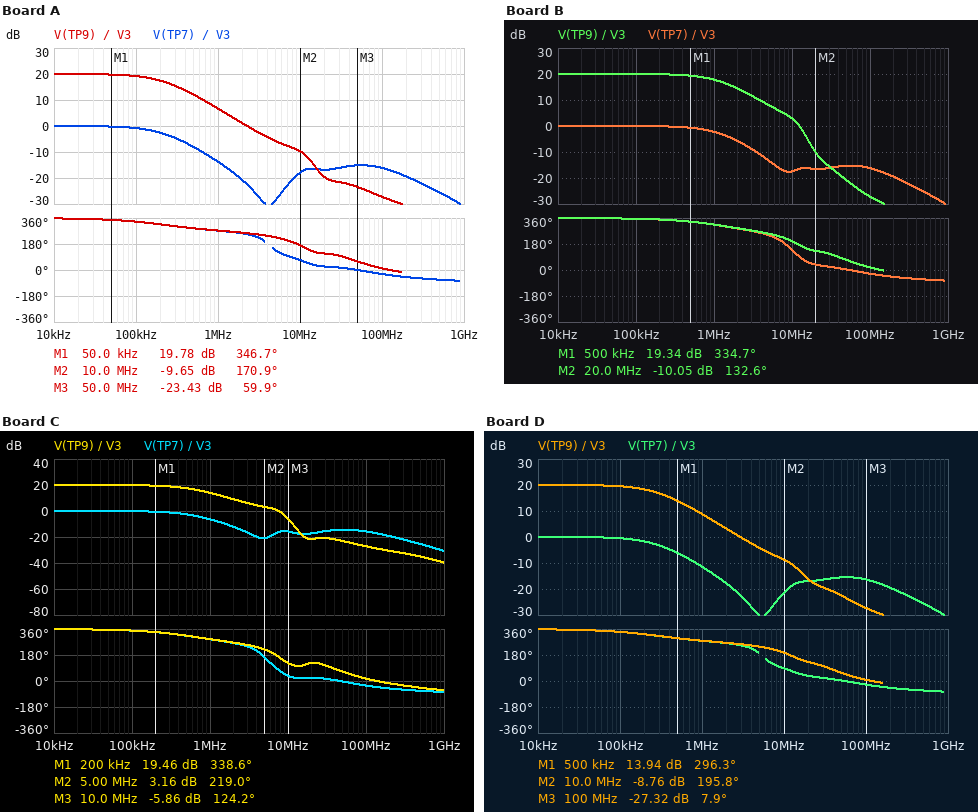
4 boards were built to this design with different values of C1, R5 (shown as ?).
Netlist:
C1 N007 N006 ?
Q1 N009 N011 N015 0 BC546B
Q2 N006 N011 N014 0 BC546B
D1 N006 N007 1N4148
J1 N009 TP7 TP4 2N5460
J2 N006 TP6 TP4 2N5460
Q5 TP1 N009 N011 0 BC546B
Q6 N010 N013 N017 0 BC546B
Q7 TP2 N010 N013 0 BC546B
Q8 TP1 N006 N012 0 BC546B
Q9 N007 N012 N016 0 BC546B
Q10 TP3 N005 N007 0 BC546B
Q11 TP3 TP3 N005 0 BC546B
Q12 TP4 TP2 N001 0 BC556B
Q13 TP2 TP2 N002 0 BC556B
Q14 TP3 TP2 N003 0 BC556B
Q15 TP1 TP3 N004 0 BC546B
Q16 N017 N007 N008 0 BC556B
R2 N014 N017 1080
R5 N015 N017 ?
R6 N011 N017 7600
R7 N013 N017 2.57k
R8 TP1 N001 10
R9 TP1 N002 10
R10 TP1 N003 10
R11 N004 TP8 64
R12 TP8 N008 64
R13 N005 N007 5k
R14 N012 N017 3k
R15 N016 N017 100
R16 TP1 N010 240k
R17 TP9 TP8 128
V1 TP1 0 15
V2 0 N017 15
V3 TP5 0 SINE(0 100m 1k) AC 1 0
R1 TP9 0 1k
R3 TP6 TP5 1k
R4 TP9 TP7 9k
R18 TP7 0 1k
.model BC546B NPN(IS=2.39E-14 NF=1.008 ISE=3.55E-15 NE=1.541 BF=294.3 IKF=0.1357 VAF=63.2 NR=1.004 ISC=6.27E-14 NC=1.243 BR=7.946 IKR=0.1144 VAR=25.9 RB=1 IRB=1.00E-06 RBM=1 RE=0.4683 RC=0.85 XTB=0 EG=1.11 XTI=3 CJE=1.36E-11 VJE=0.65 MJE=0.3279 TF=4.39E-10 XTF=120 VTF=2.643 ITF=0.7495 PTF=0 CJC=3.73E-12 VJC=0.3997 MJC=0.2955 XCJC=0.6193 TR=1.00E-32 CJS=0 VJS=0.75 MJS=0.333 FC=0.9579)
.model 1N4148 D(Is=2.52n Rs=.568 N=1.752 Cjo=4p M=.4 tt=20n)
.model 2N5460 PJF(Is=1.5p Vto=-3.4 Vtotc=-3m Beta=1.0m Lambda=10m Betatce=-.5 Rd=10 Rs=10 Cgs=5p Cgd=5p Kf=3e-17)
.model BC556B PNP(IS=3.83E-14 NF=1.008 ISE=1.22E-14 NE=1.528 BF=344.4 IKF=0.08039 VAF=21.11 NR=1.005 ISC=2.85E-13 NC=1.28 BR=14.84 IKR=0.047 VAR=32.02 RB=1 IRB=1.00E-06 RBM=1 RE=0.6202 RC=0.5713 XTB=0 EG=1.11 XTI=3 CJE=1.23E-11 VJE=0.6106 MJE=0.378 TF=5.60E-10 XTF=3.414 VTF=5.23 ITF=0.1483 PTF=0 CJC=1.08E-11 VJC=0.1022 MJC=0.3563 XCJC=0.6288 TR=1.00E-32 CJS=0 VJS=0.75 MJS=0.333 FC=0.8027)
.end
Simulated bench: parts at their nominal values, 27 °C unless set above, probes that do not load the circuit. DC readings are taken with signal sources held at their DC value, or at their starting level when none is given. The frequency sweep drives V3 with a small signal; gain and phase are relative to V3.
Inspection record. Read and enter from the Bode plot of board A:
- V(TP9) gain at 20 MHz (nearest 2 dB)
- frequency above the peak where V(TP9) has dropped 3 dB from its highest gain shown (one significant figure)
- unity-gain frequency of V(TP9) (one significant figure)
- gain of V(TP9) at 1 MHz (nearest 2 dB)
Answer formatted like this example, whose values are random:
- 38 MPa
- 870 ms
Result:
- -20 dB
- 200 kHz
- 2 MHz
- 6 dB
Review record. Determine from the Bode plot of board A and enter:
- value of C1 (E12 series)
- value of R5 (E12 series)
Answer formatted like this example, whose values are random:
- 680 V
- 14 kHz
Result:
- 56 pF
- 1.2 kΩ
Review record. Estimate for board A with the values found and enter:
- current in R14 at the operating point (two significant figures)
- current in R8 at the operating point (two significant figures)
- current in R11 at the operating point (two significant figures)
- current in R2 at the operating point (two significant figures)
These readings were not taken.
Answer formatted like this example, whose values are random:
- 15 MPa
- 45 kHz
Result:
- 210 µA
- 390 µA
- 320 µA
- 200 µA
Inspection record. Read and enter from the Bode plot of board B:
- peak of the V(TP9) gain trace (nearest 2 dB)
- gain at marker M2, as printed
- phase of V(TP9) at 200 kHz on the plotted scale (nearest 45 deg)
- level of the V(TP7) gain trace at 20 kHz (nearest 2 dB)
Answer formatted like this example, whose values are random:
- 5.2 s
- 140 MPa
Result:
- 20 dB
- -10.05 dB
- 360 deg
- 0 dB
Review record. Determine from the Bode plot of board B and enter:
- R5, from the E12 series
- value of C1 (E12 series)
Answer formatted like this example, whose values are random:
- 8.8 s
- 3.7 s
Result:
- 820 Ω
- 8.2 pF
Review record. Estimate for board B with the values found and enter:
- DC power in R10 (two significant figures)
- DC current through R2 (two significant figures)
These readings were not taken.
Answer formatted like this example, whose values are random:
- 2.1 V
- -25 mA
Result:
- 1.3 µW
- 170 µA
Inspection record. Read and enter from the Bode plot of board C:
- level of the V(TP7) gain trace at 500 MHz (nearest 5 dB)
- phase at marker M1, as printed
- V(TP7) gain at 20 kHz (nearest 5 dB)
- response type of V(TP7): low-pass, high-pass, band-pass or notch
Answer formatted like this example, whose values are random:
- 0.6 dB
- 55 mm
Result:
- -25 dB
- 338.6 deg
- 0 dB
- low-pass
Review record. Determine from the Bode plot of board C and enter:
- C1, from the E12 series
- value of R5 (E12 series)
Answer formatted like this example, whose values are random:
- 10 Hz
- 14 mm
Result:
- 39 pF
- 3.3 kΩ
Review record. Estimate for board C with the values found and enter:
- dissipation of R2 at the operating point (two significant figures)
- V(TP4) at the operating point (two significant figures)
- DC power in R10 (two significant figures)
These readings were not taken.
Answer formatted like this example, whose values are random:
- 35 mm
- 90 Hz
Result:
- 88 µW
- -2.9 V
- 1.1 µW
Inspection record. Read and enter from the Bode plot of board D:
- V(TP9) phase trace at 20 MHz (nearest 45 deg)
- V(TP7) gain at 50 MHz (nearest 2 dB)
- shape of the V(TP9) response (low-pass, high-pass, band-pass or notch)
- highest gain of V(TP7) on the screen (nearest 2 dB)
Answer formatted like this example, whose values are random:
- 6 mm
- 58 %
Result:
- 135 deg
- -16 dB
- low-pass
- 0 dB
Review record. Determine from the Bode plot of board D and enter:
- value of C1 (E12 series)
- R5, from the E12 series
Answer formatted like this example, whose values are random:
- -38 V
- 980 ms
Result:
- 33 pF
- 680 Ω
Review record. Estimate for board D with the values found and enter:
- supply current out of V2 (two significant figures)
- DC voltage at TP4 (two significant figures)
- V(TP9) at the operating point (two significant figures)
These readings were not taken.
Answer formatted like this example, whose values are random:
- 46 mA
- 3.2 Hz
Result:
- 2.3 mA
- -3.0 V
- -830 mV
